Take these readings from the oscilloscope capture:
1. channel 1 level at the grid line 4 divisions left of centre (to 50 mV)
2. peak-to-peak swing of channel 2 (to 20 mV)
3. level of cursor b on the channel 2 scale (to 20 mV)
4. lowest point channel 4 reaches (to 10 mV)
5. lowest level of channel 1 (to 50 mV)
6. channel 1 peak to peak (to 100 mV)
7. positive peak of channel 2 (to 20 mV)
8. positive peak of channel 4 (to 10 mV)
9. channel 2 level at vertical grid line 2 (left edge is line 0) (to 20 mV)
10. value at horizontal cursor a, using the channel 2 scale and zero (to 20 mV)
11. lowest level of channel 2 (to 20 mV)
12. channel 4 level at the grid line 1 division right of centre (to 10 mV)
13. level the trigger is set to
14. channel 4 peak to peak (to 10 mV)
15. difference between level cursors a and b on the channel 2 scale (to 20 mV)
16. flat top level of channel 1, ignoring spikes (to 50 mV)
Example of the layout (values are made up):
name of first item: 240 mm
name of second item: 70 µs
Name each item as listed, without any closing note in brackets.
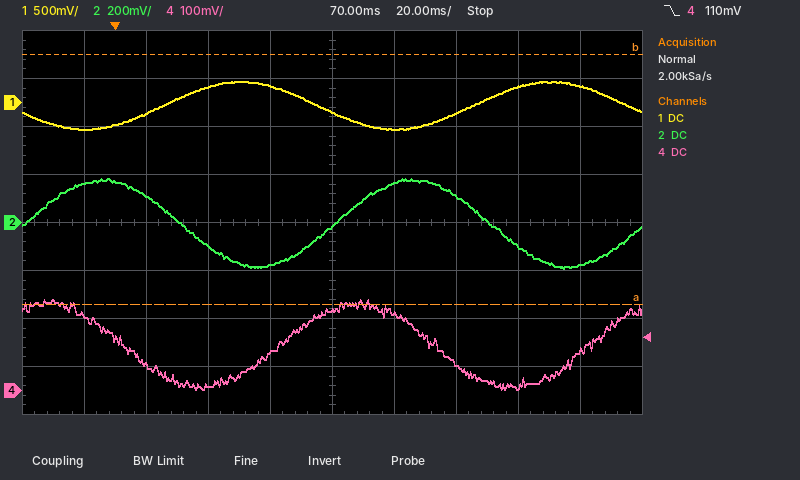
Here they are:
channel 1 level at the grid line 4 divisions left of centre: -300 mV
peak-to-peak swing of channel 2: 380 mV
level of cursor b on the channel 2 scale: 700 mV
lowest point channel 4 reaches: 0 mV
lowest level of channel 1: -300 mV
channel 1 peak to peak: 500 mV
positive peak of channel 2: 180 mV
positive peak of channel 4: 190 mV
channel 2 level at vertical grid line 2 (left edge is line 0): 120 mV
value at horizontal cursor a, using the channel 2 scale and zero: -340 mV
lowest level of channel 2: -200 mV
channel 4 level at the grid line 1 division right of centre: 160 mV
level the trigger is set to: 110 mV
channel 4 peak to peak: 190 mV
difference between level cursors a and b on the channel 2 scale: 1.04 V
flat top level of channel 1, ignoring spikes: 200 mV
